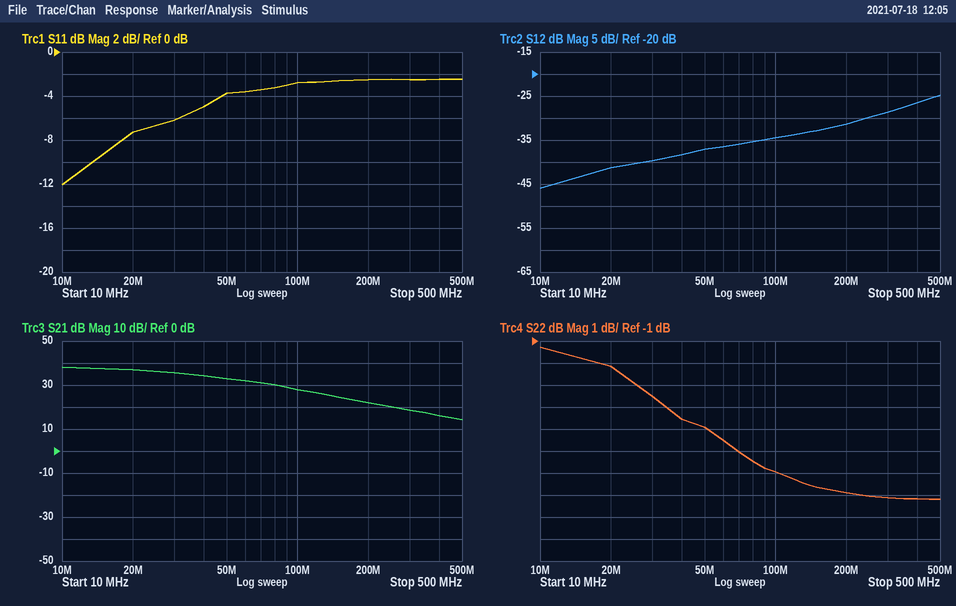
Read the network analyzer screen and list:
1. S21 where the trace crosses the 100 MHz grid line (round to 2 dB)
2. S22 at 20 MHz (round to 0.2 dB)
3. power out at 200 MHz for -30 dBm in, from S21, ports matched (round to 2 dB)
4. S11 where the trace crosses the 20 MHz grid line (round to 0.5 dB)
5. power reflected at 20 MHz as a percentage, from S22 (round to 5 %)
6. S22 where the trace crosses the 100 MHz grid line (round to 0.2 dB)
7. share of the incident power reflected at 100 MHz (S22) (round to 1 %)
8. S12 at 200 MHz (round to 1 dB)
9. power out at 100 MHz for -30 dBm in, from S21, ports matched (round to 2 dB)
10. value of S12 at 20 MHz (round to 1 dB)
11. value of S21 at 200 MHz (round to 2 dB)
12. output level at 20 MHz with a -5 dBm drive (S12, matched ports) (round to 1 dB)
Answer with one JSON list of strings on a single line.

["28 dB", "-2.2 dB", "-8 dBm", "-7.5 dB", "60 %", "-7.0 dB", "20 %", "-31 dB", "-2 dBm", "-41 dB", "22 dB", "-46 dBm"]
